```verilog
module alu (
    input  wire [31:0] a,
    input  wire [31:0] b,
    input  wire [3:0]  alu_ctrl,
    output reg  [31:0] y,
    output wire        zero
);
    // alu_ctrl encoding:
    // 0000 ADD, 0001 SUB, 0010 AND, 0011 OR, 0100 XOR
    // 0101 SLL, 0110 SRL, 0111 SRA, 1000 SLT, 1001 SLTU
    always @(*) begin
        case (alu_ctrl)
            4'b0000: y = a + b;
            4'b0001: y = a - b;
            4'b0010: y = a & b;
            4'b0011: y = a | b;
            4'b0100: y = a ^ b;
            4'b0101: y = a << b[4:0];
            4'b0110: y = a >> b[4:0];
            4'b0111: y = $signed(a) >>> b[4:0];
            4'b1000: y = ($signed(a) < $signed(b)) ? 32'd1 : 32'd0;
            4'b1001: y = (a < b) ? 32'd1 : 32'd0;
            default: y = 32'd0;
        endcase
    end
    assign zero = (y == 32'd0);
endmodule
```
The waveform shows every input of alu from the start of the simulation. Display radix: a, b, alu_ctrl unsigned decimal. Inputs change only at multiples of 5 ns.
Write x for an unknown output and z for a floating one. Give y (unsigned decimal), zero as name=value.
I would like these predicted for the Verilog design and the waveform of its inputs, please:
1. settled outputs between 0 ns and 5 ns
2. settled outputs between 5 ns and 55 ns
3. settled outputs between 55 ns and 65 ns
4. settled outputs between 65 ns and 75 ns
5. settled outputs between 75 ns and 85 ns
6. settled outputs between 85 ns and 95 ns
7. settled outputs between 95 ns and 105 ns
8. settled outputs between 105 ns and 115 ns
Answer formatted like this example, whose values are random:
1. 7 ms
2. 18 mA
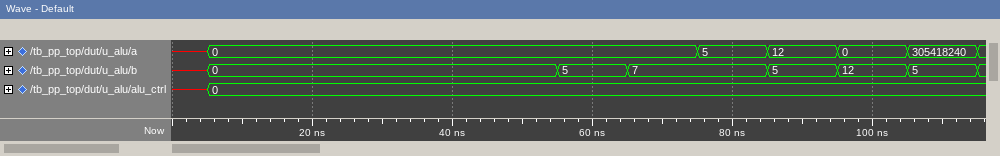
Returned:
1. y=x, zero=x
2. y=0, zero=1
3. y=5, zero=0
4. y=7, zero=0
5. y=12, zero=0
6. y=17, zero=0
7. y=12, zero=0
8. y=305418245, zero=0
